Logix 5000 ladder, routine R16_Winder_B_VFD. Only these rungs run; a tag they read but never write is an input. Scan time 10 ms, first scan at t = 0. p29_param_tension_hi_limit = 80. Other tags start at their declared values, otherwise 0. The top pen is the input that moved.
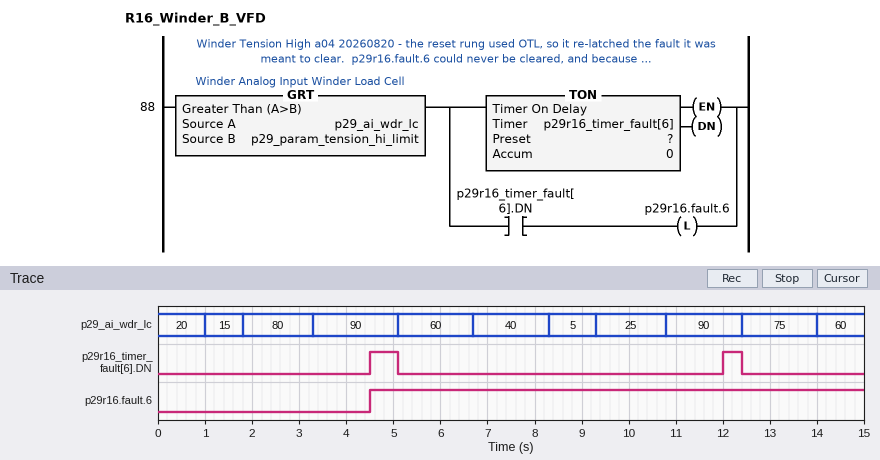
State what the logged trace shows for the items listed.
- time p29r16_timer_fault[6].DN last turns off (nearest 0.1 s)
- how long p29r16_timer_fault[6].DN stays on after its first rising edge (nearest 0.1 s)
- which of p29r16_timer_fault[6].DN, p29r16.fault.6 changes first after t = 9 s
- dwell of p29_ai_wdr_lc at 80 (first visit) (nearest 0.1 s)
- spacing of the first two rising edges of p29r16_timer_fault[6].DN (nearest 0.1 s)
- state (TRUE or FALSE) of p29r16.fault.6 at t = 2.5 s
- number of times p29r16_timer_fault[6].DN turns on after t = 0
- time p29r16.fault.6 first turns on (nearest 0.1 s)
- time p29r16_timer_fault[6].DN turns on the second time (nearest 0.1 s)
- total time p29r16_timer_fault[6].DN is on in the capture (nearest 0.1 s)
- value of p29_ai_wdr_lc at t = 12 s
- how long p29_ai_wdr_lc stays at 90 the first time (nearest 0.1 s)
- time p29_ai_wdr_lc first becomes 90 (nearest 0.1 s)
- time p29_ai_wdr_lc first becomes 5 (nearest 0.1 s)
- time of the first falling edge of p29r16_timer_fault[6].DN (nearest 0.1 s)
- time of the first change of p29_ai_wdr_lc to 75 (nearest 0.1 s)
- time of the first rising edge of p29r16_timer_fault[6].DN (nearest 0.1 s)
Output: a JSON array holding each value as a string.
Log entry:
["12.4 s", "0.6 s", "p29r16_timer_fault[6].DN", "1.5 s", "7.5 s", "FALSE", "2", "4.5 s", "12.0 s", "1.0 s", "90", "1.8 s", "3.3 s", "8.3 s", "5.1 s", "12.4 s", "4.5 s"]
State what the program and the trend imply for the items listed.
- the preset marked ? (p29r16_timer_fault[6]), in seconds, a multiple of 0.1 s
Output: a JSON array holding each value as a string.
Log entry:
["1.2 s"]
